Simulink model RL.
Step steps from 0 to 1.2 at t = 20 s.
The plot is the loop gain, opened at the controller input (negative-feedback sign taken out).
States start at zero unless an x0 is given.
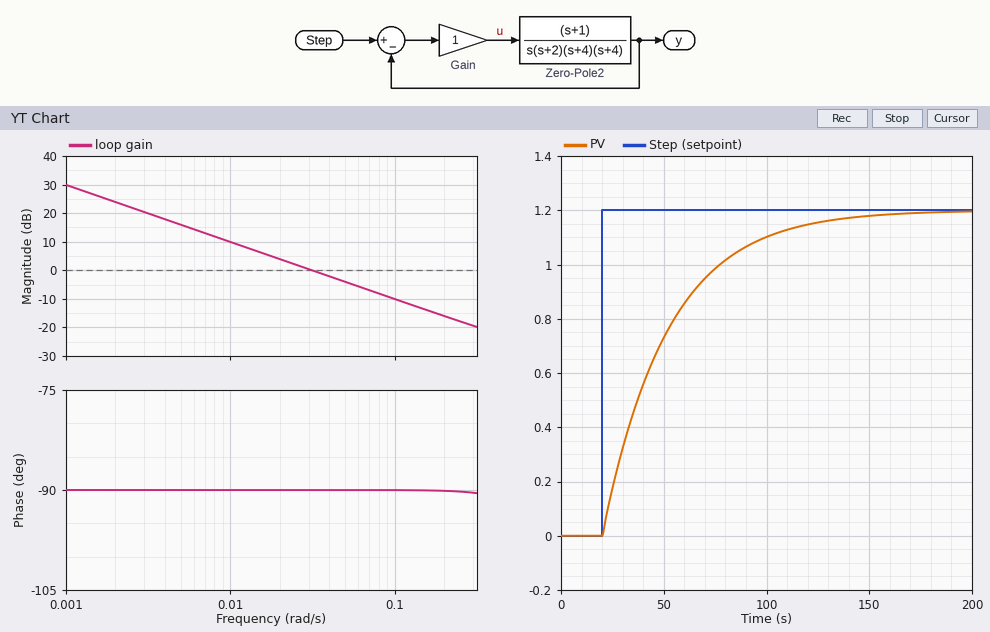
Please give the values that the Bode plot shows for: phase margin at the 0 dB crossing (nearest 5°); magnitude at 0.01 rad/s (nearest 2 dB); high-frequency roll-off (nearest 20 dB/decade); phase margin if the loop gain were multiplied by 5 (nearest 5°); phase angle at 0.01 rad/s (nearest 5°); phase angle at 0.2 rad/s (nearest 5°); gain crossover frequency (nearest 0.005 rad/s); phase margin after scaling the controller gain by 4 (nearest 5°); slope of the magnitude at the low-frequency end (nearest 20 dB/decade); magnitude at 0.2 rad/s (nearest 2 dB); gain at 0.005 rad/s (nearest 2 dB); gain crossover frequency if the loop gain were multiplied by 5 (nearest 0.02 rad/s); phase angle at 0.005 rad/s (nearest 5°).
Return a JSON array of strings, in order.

["90°", "10 dB", "-20 dB/decade", "90°", "-90°", "-90°", "0.030 rad/s", "90°", "-20 dB/decade", "-16 dB", "16 dB", "0.16 rad/s", "-90°"]
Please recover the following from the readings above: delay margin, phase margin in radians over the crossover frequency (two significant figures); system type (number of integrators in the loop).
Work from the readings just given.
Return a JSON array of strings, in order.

["52 s", "1"]
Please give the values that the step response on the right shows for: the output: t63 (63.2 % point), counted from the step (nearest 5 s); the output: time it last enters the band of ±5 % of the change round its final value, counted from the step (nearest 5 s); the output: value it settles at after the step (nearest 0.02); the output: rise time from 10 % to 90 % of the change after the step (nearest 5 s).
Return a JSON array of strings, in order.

["30 s", "95 s", "1.20", "70 s"]
